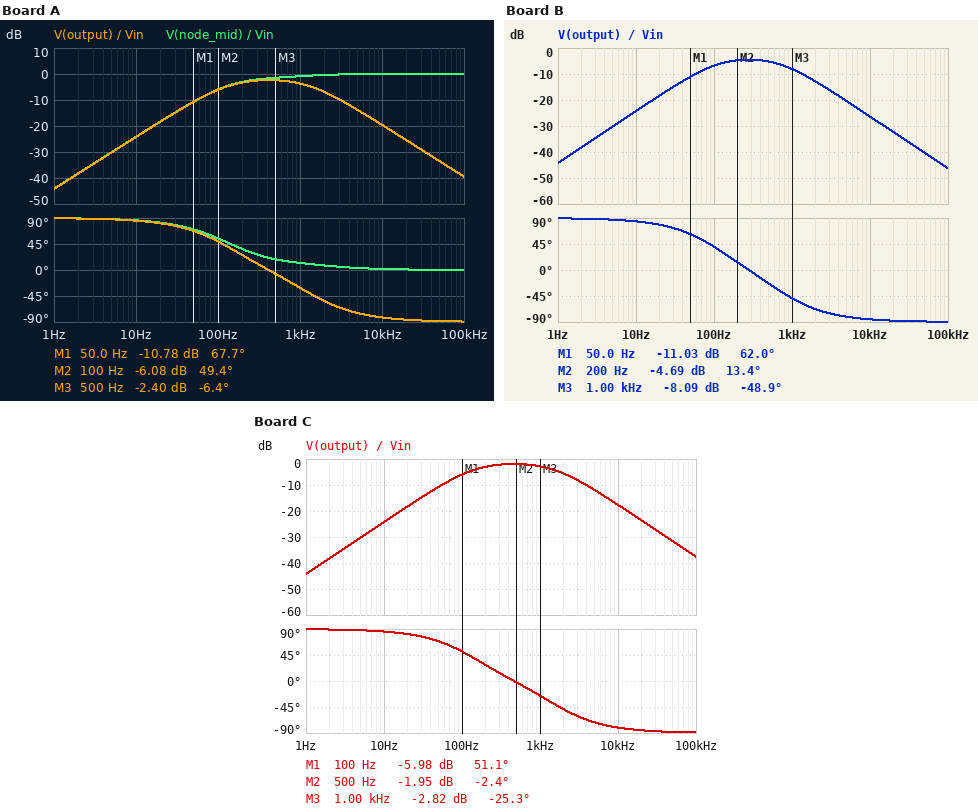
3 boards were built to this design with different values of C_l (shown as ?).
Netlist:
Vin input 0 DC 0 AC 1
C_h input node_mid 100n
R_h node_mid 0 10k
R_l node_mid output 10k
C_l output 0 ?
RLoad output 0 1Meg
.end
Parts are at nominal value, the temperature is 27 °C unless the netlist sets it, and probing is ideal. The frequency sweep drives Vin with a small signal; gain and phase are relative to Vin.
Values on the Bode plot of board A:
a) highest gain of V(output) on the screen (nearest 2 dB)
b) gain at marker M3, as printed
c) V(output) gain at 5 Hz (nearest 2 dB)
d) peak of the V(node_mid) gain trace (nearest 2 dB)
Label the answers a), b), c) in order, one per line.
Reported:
a) -2 dB
b) -2.40 dB
c) -30 dB
d) 0 dB
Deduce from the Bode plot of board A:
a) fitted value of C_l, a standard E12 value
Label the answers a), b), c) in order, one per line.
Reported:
a) 15 nF
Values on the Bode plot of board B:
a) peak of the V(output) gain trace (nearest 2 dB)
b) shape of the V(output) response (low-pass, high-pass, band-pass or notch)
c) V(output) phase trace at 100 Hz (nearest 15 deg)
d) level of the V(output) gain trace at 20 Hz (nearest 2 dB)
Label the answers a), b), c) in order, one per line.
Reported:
a) -4 dB
b) band-pass
c) 45 deg
d) -18 dB
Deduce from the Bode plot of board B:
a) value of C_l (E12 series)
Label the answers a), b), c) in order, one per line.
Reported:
a) 33 nF
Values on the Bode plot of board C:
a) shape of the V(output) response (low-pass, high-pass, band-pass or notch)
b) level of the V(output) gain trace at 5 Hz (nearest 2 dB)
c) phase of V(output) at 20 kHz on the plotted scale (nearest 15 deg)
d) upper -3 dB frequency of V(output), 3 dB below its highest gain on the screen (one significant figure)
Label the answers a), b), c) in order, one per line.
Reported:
a) band-pass
b) -30 dB
c) -90 deg
d) 2 kHz
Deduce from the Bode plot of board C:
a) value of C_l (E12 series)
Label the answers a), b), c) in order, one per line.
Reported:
a) 12 nF
